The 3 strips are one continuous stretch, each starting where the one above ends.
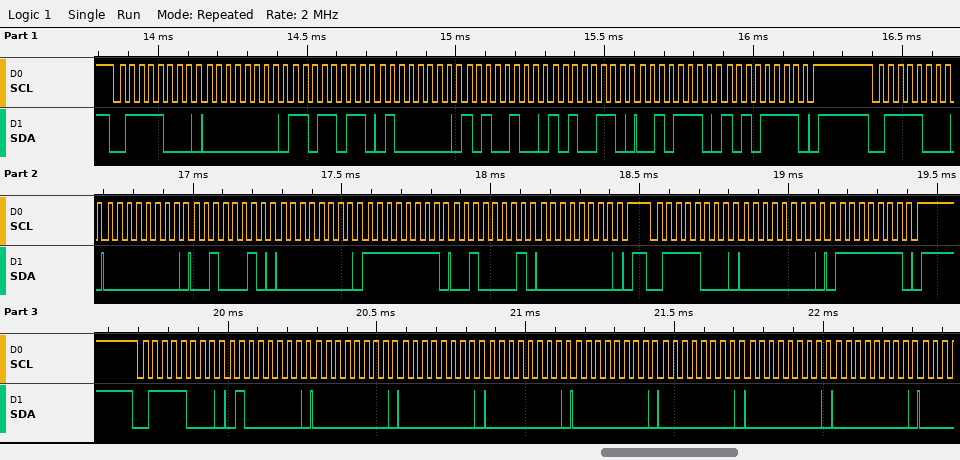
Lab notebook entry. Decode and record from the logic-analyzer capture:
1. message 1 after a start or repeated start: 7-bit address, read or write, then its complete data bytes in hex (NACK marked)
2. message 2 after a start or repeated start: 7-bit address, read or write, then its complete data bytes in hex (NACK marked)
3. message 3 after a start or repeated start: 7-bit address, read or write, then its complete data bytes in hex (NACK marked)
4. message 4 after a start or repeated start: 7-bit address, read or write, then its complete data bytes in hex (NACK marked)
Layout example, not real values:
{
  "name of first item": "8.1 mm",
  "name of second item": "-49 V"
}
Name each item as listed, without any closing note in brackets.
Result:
{
  "message 1 after a start or repeated start: 7-bit address, read or write, then its complete data bytes in hex": "0x3C write: 00 DB 40 A4 A6 2E AF",
  "message 2 after a start or repeated start: 7-bit address, read or write, then its complete data bytes in hex": "0x3C write: 00 22 00 FF 21 00",
  "message 3 after a start or repeated start: 7-bit address, read or write, then its complete data bytes in hex": "0x3C write: 00 7F",
  "message 4 after a start or repeated start: 7-bit address, read or write, then its complete data bytes in hex": "0x3C write: 40 00 00 00 00 00 00 00"
}
